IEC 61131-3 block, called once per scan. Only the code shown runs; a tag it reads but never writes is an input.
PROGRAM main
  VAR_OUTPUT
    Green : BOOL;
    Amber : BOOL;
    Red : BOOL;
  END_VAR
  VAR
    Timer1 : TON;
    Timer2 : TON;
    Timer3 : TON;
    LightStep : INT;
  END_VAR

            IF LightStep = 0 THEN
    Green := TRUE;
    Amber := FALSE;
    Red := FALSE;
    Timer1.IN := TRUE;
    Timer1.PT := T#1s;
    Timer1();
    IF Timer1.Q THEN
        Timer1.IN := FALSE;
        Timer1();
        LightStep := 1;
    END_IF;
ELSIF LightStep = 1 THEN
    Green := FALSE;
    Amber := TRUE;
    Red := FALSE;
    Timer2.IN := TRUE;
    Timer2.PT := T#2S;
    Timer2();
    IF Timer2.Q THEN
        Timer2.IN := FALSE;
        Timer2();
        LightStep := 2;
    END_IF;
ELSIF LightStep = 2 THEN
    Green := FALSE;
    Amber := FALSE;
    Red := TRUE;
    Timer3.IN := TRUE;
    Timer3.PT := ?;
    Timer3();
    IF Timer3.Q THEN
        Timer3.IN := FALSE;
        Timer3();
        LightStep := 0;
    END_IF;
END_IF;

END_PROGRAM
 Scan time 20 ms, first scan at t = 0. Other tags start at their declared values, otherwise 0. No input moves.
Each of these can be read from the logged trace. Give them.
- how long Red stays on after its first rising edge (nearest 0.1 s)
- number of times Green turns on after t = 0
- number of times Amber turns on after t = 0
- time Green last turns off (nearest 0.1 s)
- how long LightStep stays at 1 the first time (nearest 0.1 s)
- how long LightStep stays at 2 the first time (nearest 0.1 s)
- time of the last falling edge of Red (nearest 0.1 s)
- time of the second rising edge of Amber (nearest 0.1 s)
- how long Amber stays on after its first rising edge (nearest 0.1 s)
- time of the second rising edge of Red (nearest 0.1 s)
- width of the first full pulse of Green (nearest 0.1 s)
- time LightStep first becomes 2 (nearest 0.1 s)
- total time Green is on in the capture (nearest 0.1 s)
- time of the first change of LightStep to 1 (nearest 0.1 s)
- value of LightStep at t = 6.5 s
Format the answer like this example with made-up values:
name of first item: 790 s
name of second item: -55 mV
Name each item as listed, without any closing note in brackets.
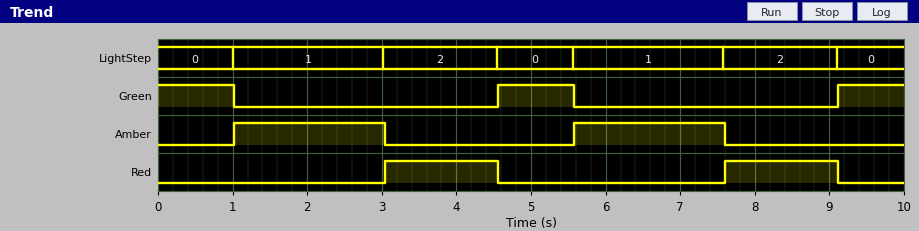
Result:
how long Red stays on after its first rising edge: 1.5 s
number of times Green turns on after t = 0: 2
number of times Amber turns on after t = 0: 2
time Green last turns off: 5.6 s
how long LightStep stays at 1 the first time: 2.0 s
how long LightStep stays at 2 the first time: 1.5 s
time of the last falling edge of Red: 9.1 s
time of the second rising edge of Amber: 5.6 s
how long Amber stays on after its first rising edge: 2.0 s
time of the second rising edge of Red: 7.6 s
width of the first full pulse of Green: 1.0 s
time LightStep first becomes 2: 3.0 s
total time Green is on in the capture: 2.9 s
time of the first change of LightStep to 1: 1.0 s
value of LightStep at t = 6.5 s: 1
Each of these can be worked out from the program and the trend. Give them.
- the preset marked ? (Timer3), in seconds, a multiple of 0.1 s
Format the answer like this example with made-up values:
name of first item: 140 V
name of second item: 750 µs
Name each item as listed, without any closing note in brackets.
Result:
the preset marked ? (Timer3), in seconds, a multiple of 0.1 s: 1.5 s
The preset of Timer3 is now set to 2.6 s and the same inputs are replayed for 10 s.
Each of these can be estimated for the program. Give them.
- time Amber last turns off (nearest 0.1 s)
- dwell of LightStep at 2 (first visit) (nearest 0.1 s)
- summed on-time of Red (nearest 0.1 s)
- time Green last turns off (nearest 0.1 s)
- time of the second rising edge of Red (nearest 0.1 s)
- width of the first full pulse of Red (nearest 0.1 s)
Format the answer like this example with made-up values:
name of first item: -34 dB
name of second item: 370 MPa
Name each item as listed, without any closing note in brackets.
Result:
time Amber last turns off: 8.7 s
dwell of LightStep at 2 (first visit): 2.6 s
summed on-time of Red: 3.9 s
time Green last turns off: 6.7 s
time of the second rising edge of Red: 8.7 s
width of the first full pulse of Red: 2.6 s
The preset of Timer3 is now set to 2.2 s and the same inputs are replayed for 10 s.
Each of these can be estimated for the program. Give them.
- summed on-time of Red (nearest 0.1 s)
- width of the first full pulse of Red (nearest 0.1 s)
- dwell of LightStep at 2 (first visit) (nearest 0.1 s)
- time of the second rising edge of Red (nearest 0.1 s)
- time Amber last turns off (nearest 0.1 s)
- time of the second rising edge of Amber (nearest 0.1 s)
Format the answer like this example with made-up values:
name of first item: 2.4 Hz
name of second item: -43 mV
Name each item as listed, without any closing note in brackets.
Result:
summed on-time of Red: 3.9 s
width of the first full pulse of Red: 2.2 s
dwell of LightStep at 2 (first visit): 2.2 s
time of the second rising edge of Red: 8.3 s
time Amber last turns off: 8.3 s
time of the second rising edge of Amber: 6.3 s
